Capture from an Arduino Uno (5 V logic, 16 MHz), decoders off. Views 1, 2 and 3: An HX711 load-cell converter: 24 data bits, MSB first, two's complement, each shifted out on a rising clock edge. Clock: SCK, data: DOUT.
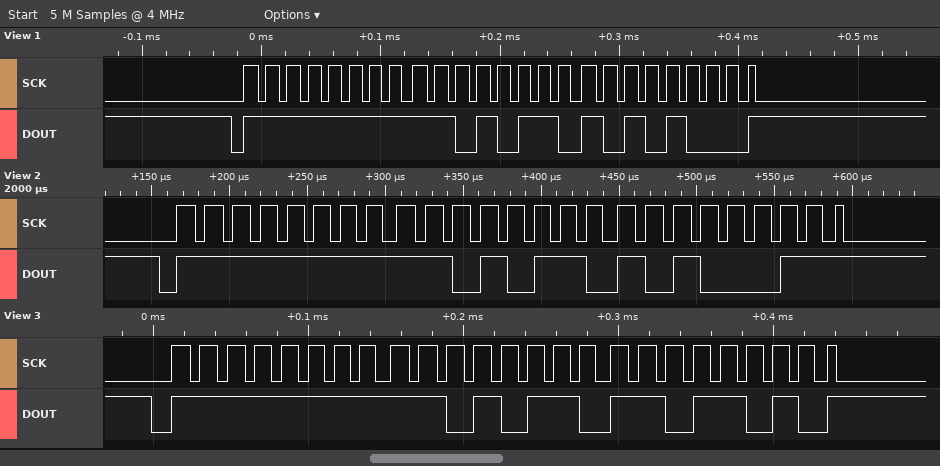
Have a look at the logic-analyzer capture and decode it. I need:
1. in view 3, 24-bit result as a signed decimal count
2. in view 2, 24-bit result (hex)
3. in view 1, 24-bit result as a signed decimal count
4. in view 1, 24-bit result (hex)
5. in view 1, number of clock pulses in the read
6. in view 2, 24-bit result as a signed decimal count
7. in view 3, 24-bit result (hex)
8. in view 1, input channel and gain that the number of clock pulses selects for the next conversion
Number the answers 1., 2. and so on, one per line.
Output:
1. -10534
2. 0xFFD6A3
3. -10584
4. 0xFFD6A8
5. 25
6. -10589
7. 0xFFD6DA
8. channel A, gain 128
